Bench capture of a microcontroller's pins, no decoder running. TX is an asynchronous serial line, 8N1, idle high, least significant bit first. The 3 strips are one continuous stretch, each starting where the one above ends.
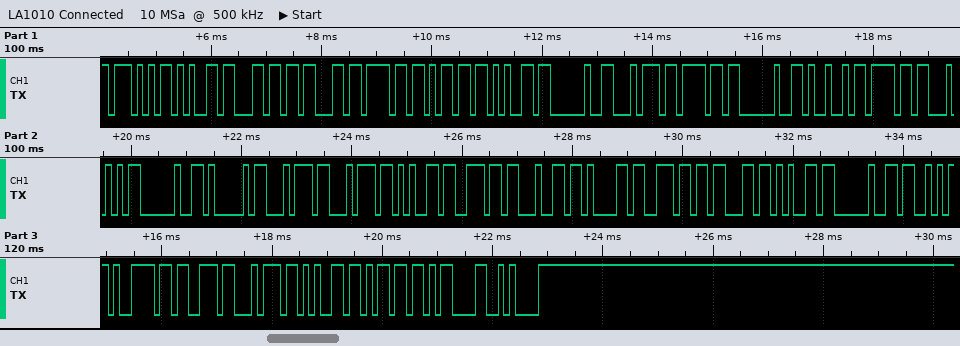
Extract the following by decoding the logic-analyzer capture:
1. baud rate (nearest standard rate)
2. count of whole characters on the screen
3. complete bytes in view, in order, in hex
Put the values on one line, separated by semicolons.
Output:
9600 baud; 34; 57 65 6C 63 6F 6D 65 20 74 6F 20 49 6F 54 20 41 74 74 65 6E 64 61 6E 63 65 20 53 79 73 74 65 6D 0D 0A
